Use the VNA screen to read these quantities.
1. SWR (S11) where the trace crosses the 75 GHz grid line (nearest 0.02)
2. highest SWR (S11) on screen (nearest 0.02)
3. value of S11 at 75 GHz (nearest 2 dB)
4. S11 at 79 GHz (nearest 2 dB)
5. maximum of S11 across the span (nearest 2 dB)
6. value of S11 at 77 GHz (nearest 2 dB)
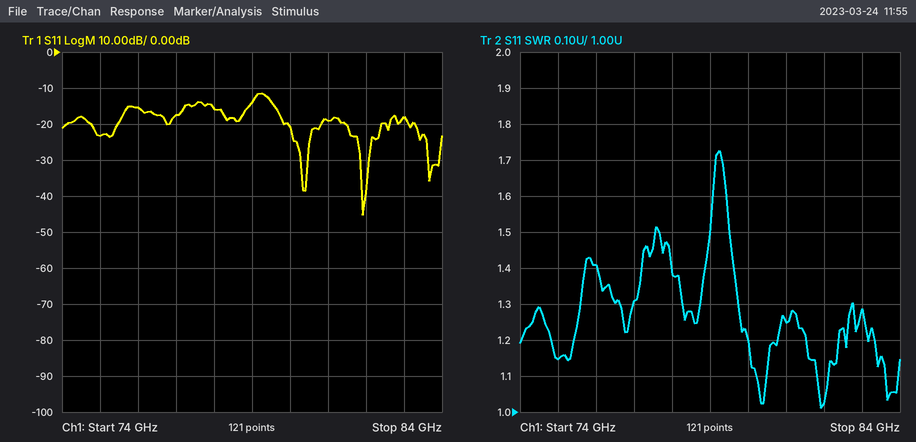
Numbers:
1.14
1.72
-24 dB
-14 dB
-12 dB
-18 dB
